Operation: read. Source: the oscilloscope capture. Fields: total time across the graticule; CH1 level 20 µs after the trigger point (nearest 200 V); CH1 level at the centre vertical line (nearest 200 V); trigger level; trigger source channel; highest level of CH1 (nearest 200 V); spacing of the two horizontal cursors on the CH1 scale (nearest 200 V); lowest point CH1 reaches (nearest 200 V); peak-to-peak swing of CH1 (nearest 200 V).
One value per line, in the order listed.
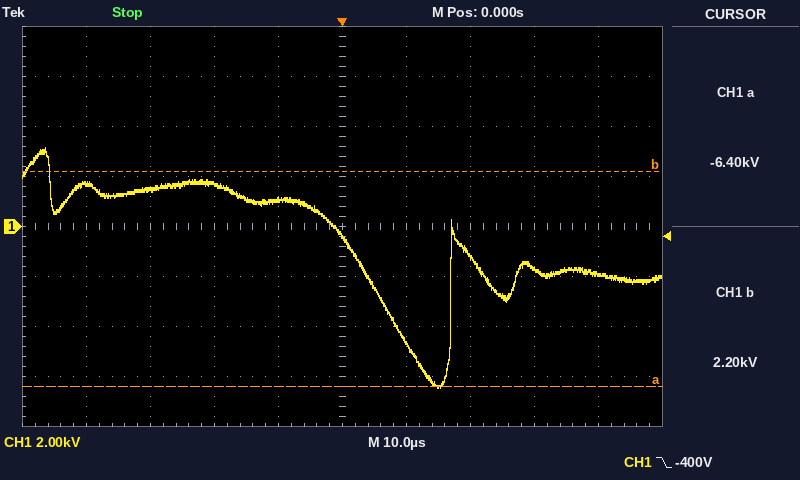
100 µs
-1.2 kV
-400 V
-400 V
CH1
3.2 kV
8.6 kV
-6.4 kV
9.6 kV
